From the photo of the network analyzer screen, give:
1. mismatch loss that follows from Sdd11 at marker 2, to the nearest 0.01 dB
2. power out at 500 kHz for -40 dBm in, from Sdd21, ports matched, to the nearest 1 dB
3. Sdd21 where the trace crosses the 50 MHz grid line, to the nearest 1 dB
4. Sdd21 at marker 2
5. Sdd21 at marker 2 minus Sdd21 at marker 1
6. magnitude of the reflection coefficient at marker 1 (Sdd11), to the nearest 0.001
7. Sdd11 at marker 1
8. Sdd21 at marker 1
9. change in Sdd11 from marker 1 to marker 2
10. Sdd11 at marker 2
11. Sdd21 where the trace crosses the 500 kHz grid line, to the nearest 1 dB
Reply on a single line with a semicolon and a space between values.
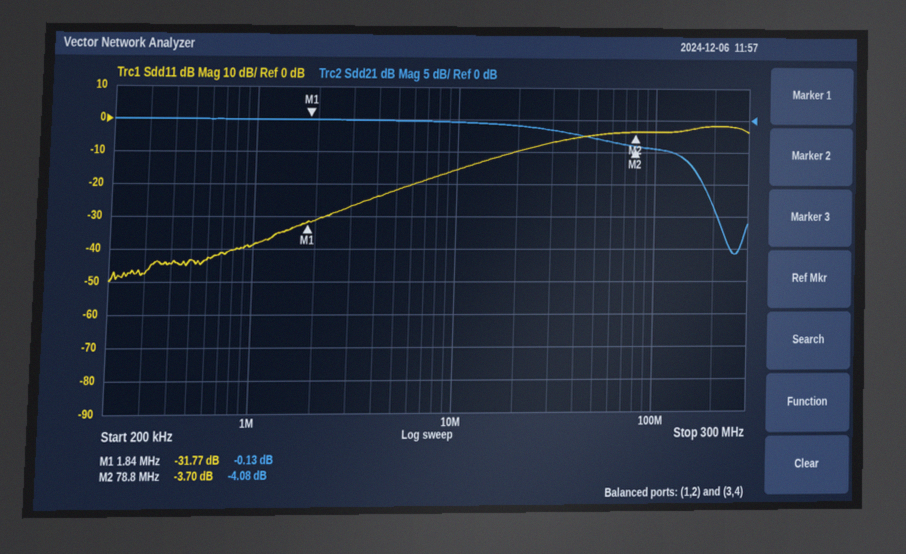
2.42 dB; -40 dBm; -3 dB; -4.08 dB; -3.95 dB; 0.026; -31.77 dB; -0.13 dB; 28.07 dB; -3.70 dB; 0 dB
